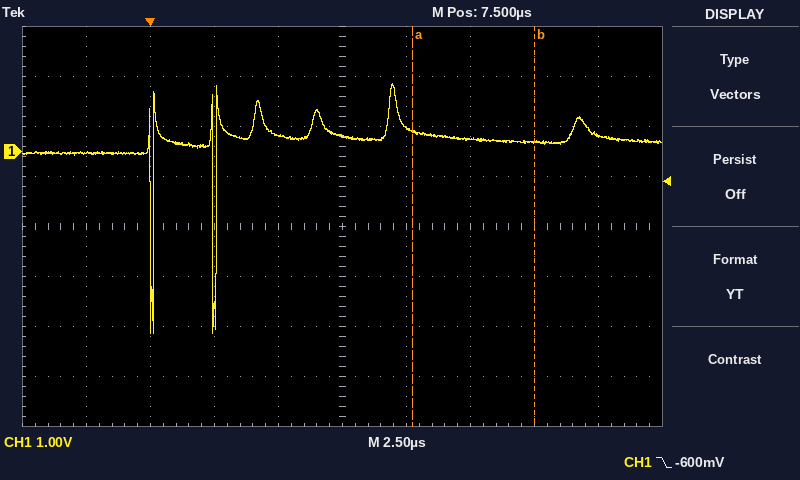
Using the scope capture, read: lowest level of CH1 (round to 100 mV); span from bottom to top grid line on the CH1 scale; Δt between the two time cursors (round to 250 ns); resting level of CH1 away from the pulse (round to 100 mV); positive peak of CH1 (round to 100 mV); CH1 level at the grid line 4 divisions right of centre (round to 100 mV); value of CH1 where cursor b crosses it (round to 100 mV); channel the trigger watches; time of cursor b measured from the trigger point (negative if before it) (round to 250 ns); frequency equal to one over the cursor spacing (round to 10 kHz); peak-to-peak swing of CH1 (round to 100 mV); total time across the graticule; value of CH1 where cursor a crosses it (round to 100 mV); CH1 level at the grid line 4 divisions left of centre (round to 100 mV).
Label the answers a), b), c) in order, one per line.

a) -3.6 V
b) 8 V
c) 4.75 µs
d) 200 mV
e) 1.4 V
f) 300 mV
g) 200 mV
h) CH1
i) +15.00 µs
j) 210 kHz
k) 5.0 V
l) 25 µs
m) 400 mV
n) 0.0 V
